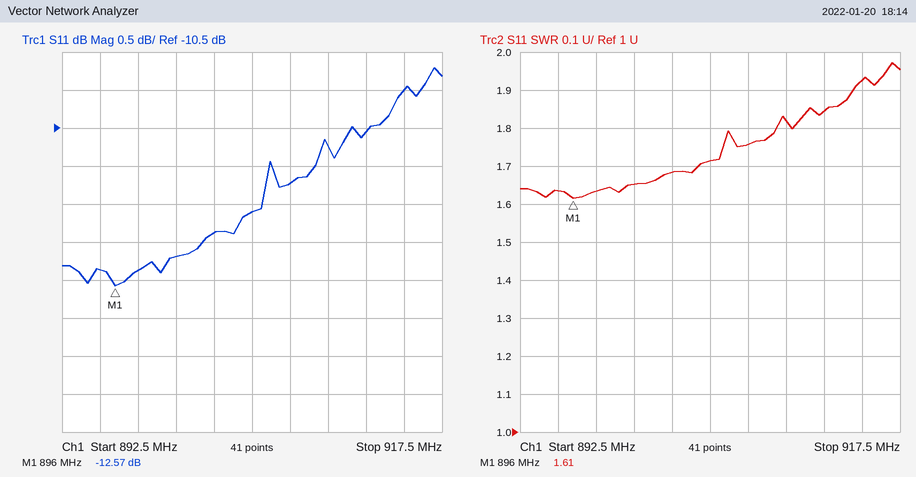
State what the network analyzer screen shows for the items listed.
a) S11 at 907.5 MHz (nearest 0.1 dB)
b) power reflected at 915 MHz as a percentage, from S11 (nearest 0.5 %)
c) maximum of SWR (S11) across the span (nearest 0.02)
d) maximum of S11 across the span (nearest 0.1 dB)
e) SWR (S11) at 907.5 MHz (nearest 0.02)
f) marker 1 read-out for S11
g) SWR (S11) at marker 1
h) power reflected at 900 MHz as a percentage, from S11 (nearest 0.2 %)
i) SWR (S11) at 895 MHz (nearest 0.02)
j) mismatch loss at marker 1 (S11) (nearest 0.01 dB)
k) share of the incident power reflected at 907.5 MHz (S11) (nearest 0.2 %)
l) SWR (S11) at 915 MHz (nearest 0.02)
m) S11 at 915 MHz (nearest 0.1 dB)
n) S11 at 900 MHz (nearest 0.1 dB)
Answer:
-11.2 dB
10.0 %
1.98
-9.7 dB
1.76
-12.57 dB
1.61
6.0 %
1.64
0.25 dB
7.6 %
1.92
-10.0 dB
-12.2 dB
